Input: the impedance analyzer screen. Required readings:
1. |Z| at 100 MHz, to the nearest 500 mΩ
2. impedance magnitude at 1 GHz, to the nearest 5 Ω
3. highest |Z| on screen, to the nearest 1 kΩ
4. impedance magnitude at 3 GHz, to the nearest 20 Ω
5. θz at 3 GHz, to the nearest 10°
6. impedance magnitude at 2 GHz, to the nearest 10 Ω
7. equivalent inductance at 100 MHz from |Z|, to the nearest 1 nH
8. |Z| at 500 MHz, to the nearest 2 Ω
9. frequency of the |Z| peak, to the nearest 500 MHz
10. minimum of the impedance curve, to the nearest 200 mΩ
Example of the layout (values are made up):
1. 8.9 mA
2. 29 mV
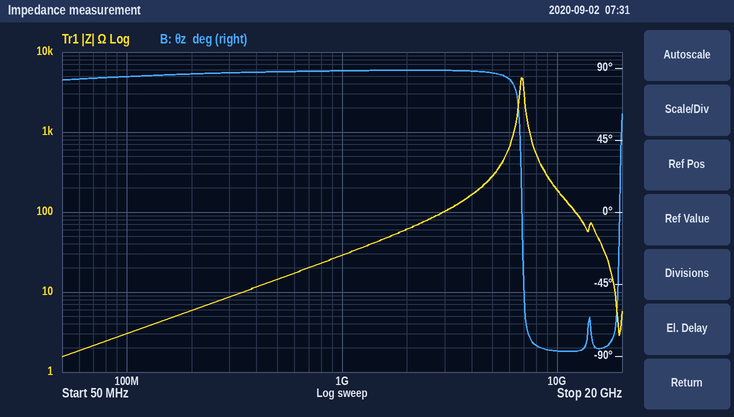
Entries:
1. 3.0 Ω
2. 30 Ω
3. 5 kΩ
4. 100 Ω
5. 90°
6. 60 Ω
7. 5 nH
8. 14 Ω
9. 7.0 GHz
10. 1.6 Ω
